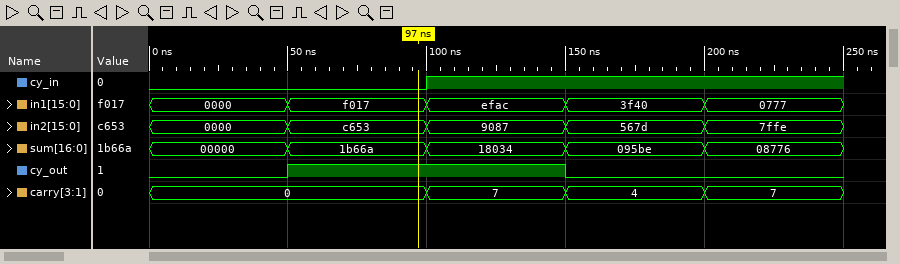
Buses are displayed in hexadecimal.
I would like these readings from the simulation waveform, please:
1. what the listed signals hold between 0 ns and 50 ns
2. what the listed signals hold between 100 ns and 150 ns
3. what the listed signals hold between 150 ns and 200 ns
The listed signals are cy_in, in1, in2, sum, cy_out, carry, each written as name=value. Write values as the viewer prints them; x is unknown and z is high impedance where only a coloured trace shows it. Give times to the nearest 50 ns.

cy_in=0, in1=0000, in2=0000, sum=00000, cy_out=0, carry=0
cy_in=1, in1=efac, in2=9087, sum=18034, cy_out=1, carry=7
cy_in=1, in1=3f40, in2=567d, sum=095be, cy_out=0, carry=4
